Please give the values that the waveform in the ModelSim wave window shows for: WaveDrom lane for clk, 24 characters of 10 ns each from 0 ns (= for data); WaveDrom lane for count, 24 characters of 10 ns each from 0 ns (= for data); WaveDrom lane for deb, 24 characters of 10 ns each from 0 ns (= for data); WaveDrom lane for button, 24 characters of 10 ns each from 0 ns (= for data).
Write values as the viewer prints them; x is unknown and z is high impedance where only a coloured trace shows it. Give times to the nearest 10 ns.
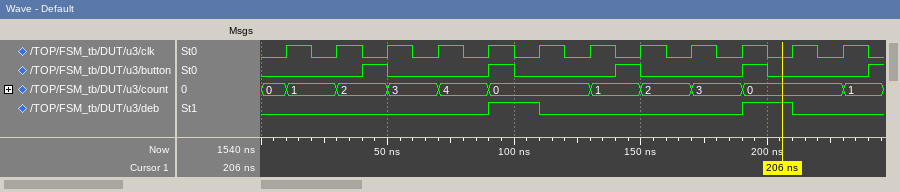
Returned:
{name: 'clk', wave: '010101010101010101010101'}
{name: 'count', wave: '==.=.=.=.=...=.=.=.=...=', data: '0 1 2 3 4 0 1 2 3 0 1'}
{name: 'deb', wave: '0........1.0.......1.0..'}
{name: 'button', wave: '0...10...10...10...10...'}
